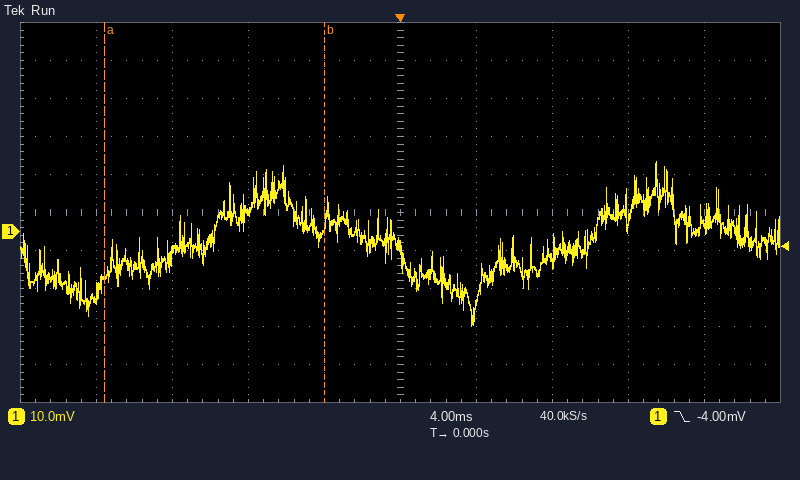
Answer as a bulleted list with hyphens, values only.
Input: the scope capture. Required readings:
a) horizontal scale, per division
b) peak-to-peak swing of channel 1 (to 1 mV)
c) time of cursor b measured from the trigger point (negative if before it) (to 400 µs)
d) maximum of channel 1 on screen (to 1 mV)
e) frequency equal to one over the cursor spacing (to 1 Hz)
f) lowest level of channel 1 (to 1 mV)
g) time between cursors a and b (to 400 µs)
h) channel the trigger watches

- 4 ms
- 43 mV
- -4.0 ms
- 18 mV
- 86 Hz
- -25 mV
- 11.6 ms
- channel 1
